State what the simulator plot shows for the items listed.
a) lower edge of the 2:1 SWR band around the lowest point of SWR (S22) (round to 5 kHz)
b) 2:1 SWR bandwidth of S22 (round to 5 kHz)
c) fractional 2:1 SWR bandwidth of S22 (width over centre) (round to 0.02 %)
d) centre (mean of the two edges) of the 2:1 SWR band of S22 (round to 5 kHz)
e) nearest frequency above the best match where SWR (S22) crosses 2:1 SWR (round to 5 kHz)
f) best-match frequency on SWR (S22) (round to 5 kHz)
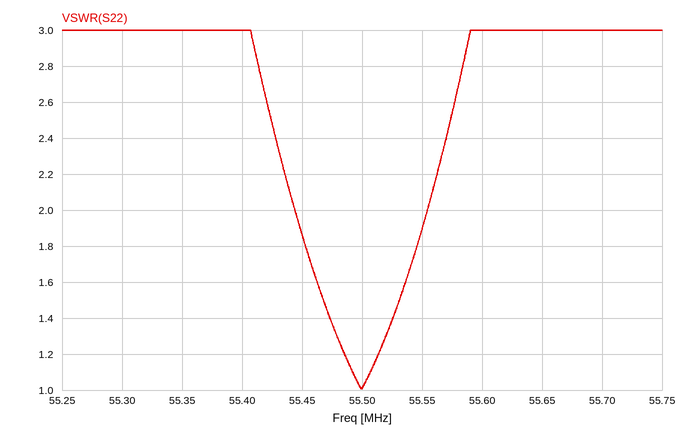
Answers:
55.445 MHz
110 kHz
0.20 %
55.500 MHz
55.555 MHz
55.500 MHz
